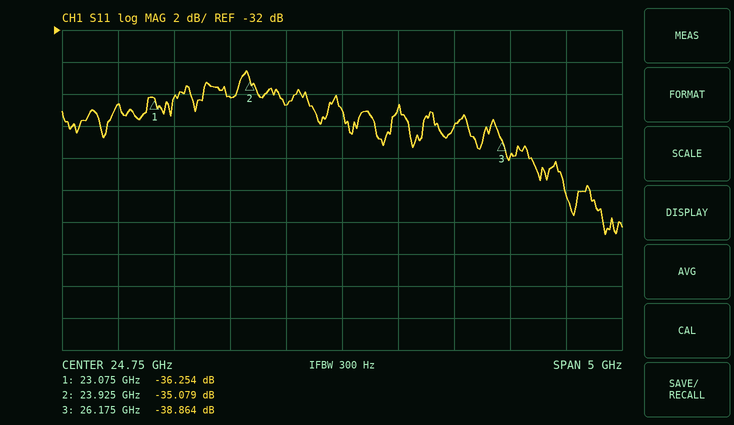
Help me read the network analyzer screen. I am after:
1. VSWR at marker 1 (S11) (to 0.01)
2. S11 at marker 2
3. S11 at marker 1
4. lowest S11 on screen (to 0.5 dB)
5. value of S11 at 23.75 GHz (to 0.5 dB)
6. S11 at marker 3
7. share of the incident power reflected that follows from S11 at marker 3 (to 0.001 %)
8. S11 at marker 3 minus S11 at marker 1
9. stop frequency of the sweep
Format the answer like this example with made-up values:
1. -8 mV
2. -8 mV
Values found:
1. 1.03
2. -35.079 dB
3. -36.254 dB
4. -45.0 dB
5. -36.0 dB
6. -38.864 dB
7. 0.013 %
8. -2.610 dB
9. 27.25 GHz
